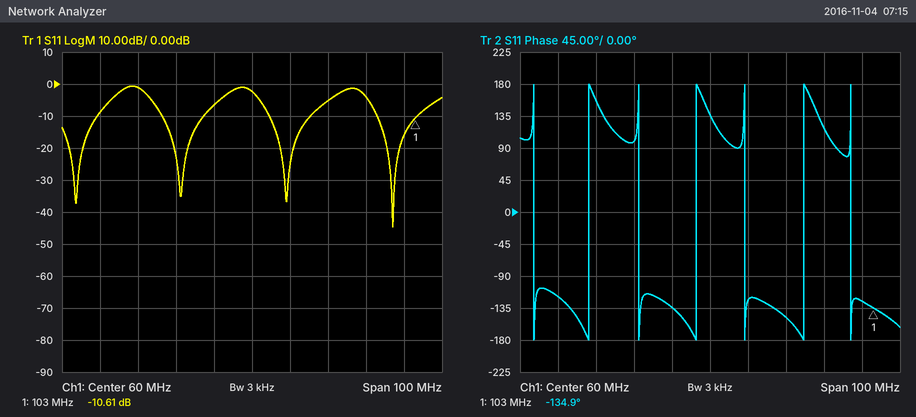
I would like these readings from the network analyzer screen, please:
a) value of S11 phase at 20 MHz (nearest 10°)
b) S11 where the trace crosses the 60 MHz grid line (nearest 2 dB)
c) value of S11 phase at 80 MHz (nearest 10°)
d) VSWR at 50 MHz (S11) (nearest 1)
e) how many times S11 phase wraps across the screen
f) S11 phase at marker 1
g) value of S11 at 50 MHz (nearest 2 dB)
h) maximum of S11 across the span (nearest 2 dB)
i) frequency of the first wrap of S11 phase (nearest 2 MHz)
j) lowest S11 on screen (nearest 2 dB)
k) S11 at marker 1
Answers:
-120°
-2 dB
-150°
3
7
-134.9°
-6 dB
0 dB
14 MHz
-44 dB
-10.61 dB
